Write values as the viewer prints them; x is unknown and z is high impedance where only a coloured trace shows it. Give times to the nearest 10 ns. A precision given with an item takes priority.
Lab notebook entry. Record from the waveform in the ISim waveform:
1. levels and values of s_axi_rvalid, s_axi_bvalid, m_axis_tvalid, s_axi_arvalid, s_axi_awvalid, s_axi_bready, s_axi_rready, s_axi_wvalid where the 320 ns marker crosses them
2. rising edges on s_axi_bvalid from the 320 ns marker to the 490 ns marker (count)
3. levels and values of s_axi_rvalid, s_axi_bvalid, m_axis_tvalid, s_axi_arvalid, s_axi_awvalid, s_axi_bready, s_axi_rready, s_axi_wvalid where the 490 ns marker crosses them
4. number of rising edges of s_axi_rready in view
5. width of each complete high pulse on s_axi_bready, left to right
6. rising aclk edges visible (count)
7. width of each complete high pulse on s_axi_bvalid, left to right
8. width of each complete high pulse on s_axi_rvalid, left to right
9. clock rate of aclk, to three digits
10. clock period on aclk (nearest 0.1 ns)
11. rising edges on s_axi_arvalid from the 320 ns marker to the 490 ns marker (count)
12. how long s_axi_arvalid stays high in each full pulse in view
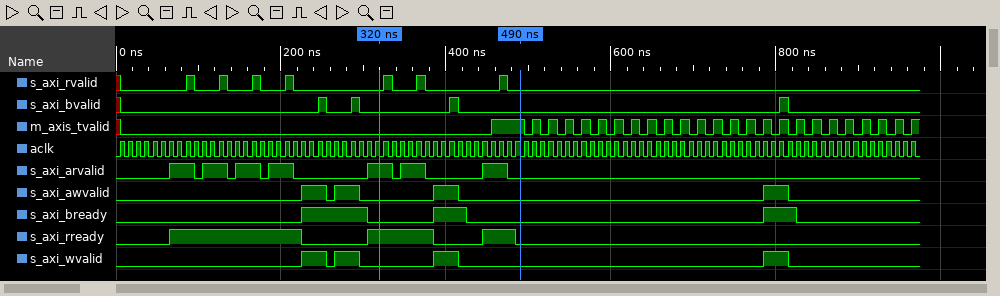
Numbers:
s_axi_rvalid=0, s_axi_bvalid=0, m_axis_tvalid=0, s_axi_arvalid=1, s_axi_awvalid=0, s_axi_bready=0, s_axi_rready=1, s_axi_wvalid=0
1
s_axi_rvalid=0, s_axi_bvalid=0, m_axis_tvalid=1, s_axi_arvalid=0, s_axi_awvalid=0, s_axi_bready=0, s_axi_rready=0, s_axi_wvalid=0
3
80 ns, 40 ns, 40 ns
97
10 ns, 10 ns, 10 ns, 10 ns
10 ns, 10 ns, 10 ns, 10 ns, 10 ns, 10 ns, 10 ns
100 MHz
10 ns
2
30 ns, 30 ns, 30 ns, 30 ns, 30 ns, 30 ns, 30 ns
